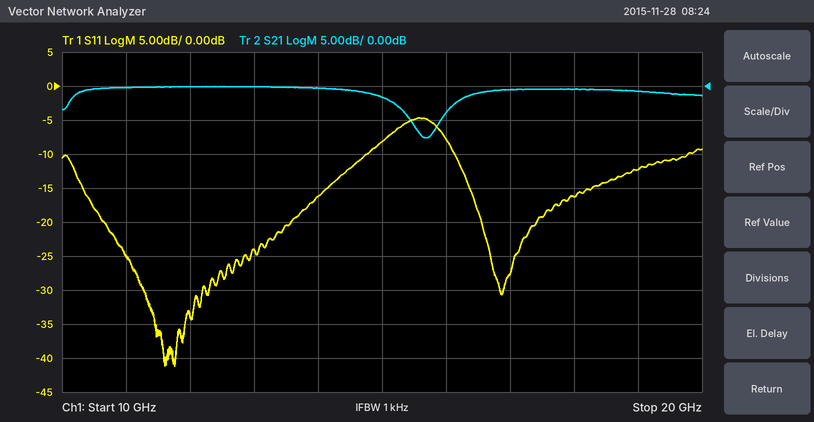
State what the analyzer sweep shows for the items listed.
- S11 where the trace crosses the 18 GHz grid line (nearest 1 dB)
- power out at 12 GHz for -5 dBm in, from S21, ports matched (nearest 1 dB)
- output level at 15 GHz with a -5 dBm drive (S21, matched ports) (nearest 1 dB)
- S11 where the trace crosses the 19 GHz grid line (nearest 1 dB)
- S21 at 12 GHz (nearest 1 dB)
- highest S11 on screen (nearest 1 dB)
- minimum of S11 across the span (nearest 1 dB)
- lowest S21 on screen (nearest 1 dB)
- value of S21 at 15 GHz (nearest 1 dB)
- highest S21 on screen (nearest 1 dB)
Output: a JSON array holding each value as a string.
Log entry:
["-16 dB", "-5 dBm", "-7 dBm", "-12 dB", "0 dB", "-5 dB", "-41 dB", "-8 dB", "-2 dB", "0 dB"]
